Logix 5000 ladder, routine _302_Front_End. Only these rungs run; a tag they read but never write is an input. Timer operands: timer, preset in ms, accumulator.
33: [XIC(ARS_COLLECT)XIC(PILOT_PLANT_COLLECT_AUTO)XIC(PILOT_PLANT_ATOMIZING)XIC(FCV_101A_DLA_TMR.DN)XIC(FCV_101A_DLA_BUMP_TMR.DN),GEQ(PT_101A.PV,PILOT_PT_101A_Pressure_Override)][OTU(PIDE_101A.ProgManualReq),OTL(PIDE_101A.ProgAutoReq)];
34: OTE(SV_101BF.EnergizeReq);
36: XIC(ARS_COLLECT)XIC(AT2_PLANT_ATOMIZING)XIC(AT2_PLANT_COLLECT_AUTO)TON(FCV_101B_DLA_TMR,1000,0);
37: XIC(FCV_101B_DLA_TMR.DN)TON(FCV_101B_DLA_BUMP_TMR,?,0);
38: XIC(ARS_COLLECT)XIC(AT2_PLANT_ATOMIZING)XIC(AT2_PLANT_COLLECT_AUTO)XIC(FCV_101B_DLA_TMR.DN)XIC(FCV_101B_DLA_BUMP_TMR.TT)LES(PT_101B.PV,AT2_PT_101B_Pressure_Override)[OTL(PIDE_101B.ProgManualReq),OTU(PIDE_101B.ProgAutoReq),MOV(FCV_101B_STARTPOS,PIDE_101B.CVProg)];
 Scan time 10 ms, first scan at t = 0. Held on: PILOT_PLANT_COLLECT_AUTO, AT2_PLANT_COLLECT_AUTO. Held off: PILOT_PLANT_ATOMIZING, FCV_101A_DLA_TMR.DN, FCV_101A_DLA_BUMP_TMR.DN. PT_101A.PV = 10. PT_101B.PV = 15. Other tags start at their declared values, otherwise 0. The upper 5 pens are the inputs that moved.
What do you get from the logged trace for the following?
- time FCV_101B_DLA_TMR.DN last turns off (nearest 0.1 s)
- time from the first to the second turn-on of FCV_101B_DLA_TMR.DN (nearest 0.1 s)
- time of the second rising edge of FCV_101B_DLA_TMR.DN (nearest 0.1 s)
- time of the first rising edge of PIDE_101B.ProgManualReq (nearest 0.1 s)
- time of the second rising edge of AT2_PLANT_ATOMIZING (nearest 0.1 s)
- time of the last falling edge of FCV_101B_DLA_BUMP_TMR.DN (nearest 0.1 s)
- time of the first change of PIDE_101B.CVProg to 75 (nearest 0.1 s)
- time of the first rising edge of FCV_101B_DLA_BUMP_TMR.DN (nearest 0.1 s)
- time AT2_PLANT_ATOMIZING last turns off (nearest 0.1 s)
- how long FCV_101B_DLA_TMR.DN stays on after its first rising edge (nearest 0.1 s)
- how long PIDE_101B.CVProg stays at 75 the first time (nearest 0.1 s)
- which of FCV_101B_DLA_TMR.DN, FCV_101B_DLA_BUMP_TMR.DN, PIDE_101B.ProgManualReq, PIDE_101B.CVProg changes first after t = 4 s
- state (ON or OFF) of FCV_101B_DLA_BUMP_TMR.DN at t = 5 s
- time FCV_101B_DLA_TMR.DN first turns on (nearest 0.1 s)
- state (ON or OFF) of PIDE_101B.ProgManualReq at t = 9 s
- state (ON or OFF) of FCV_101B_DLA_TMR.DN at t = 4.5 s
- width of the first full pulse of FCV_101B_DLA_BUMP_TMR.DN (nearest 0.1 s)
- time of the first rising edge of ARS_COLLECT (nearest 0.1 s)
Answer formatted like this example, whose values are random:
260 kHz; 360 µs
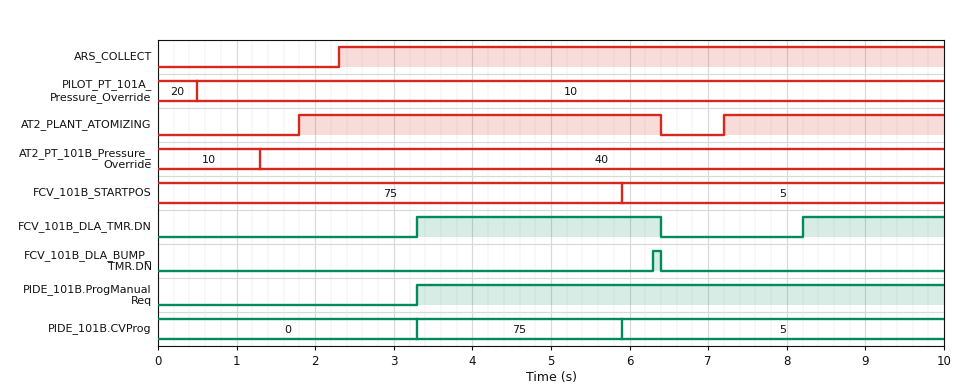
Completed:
6.4 s; 4.9 s; 8.2 s; 3.3 s; 7.2 s; 6.4 s; 3.3 s; 6.3 s; 6.4 s; 3.1 s; 2.6 s; PIDE_101B.CVProg; OFF; 3.3 s; ON; ON; 0.1 s; 2.3 s
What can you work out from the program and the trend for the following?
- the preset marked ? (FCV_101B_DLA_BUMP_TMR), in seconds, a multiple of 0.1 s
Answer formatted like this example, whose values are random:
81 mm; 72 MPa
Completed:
3.0 s
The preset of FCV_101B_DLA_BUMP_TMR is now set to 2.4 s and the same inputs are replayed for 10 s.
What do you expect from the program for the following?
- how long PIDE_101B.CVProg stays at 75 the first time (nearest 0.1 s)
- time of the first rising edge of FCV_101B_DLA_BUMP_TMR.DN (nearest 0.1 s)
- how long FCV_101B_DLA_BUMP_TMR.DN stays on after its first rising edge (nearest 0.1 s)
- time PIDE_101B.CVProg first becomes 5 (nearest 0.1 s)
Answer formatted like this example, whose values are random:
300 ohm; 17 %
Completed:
4.9 s; 5.7 s; 0.7 s; 8.2 s
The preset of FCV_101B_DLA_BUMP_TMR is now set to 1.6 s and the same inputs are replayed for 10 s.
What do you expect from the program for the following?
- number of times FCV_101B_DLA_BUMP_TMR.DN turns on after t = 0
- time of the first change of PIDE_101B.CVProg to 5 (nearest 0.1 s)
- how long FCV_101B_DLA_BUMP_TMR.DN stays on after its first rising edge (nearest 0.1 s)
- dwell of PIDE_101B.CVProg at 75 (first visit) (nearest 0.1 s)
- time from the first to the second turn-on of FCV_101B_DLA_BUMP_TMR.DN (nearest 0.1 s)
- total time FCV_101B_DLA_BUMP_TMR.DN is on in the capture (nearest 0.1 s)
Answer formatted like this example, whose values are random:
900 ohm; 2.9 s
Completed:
2; 8.2 s; 1.5 s; 4.9 s; 4.9 s; 1.7 s
